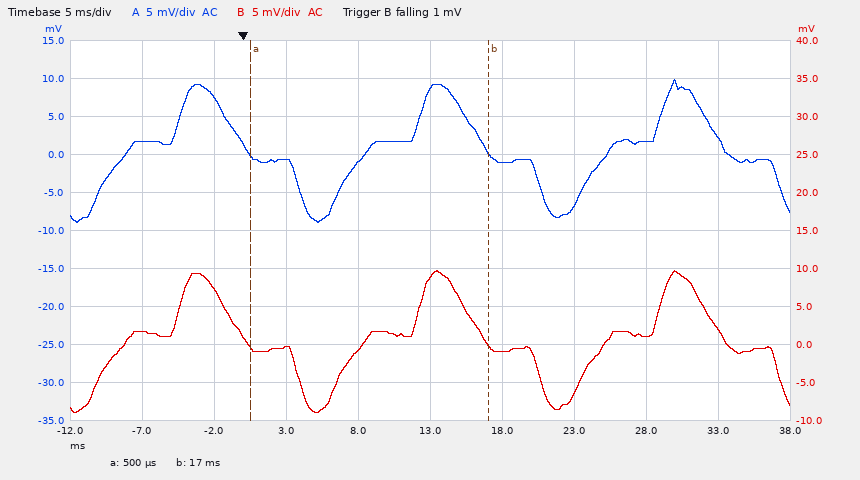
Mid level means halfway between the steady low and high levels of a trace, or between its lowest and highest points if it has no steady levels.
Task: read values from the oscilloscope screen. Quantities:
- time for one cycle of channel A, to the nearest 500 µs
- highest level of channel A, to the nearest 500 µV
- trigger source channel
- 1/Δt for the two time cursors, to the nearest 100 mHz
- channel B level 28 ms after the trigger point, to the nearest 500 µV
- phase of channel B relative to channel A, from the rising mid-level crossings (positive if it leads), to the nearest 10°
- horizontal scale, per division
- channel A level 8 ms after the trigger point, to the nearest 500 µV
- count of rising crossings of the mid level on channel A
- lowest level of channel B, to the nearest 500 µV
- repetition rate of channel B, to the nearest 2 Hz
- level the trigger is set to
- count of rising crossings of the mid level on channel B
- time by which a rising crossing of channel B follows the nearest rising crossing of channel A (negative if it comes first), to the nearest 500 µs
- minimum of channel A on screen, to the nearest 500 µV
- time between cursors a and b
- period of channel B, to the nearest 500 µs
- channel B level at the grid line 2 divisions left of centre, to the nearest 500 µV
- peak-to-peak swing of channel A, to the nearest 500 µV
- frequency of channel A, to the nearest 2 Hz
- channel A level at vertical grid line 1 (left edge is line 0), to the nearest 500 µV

16.5 ms
10.0 mV
channel B
60.6 Hz
1.0 mV
0°
5 ms
-1.0 mV
3
-9.0 mV
60 Hz
1 mV
3
0.0 ms
-9.0 mV
16.5 ms
16.5 ms
-500 µV
19.0 mV
60 Hz
1.5 mV
